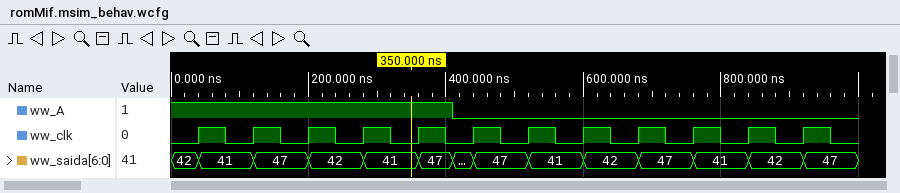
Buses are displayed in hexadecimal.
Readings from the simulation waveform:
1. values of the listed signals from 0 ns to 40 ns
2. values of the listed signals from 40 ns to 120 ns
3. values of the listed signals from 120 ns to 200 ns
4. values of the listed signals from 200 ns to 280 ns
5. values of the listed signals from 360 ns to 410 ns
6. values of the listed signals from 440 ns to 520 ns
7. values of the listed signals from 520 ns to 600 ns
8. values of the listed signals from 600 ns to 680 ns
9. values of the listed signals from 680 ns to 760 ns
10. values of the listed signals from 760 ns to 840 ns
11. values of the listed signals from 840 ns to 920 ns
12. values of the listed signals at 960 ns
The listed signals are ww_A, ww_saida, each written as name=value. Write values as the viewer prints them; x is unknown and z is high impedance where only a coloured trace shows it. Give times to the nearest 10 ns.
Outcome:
ww_A=1, ww_saida=42
ww_A=1, ww_saida=41
ww_A=1, ww_saida=47
ww_A=1, ww_saida=42
ww_A=1, ww_saida=47
ww_A=0, ww_saida=47
ww_A=0, ww_saida=41
ww_A=0, ww_saida=42
ww_A=0, ww_saida=47
ww_A=0, ww_saida=41
ww_A=0, ww_saida=42
ww_A=0, ww_saida=47
